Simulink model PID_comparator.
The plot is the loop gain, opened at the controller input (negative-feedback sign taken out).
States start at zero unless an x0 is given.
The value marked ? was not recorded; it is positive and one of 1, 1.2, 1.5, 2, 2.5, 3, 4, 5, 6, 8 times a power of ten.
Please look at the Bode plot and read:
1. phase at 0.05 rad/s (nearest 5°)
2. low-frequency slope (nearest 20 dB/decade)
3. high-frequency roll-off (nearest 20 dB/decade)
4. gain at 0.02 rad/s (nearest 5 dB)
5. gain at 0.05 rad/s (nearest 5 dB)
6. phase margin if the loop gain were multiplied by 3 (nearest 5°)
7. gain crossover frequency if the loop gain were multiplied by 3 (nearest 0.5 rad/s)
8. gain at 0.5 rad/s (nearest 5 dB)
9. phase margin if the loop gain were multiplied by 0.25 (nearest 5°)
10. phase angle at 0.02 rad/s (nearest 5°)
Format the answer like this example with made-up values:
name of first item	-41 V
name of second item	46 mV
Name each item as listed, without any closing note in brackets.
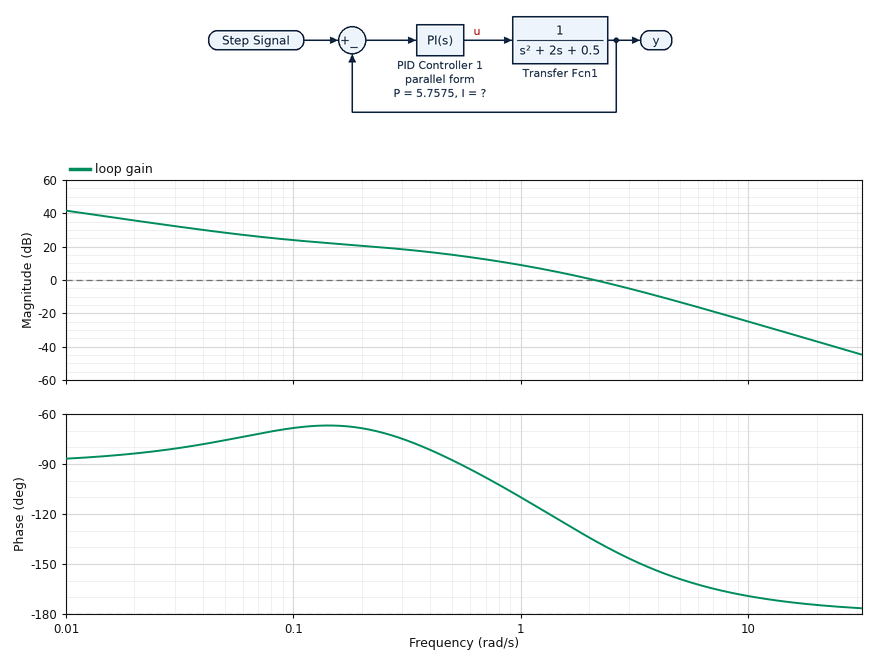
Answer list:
phase at 0.05 rad/s	-75°
low-frequency slope	-20 dB/decade
high-frequency roll-off	-40 dB/decade
gain at 0.02 rad/s	35 dB
gain at 0.05 rad/s	30 dB
phase margin if the loop gain were multiplied by 3	25°
gain crossover frequency if the loop gain were multiplied by 3	4.0 rad/s
gain at 0.5 rad/s	15 dB
phase margin if the loop gain were multiplied by 0.25	80°
phase angle at 0.02 rad/s	-85°
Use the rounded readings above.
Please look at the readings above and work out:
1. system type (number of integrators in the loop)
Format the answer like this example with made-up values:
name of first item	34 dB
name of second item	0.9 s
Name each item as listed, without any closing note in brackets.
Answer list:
system type	1
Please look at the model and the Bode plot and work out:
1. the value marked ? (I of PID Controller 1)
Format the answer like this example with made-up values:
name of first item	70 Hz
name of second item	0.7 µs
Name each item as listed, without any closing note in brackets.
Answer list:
the value marked ?	0.6
